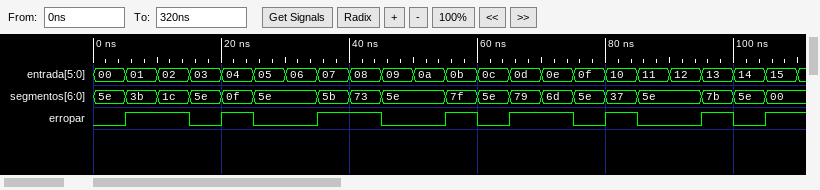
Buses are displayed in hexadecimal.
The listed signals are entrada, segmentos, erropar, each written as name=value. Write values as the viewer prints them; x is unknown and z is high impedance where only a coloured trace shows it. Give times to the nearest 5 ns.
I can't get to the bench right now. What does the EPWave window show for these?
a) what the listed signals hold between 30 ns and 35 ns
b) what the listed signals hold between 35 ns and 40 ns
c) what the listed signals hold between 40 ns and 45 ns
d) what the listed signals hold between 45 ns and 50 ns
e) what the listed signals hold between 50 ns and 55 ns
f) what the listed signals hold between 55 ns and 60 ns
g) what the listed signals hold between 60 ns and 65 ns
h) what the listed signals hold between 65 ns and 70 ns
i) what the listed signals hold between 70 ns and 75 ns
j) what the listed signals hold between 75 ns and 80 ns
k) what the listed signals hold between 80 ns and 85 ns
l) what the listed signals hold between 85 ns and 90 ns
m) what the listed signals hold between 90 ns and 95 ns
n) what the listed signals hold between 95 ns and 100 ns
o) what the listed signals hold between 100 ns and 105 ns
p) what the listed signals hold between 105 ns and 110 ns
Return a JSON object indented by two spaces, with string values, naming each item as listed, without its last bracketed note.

{
  "what the listed signals hold between 30 ns and 35 ns": "entrada=06, segmentos=5e, erropar=0",
  "what the listed signals hold between 35 ns and 40 ns": "entrada=07, segmentos=5b, erropar=1",
  "what the listed signals hold between 40 ns and 45 ns": "entrada=08, segmentos=73, erropar=1",
  "what the listed signals hold between 45 ns and 50 ns": "entrada=09, segmentos=5e, erropar=0",
  "what the listed signals hold between 50 ns and 55 ns": "entrada=0a, segmentos=5e, erropar=0",
  "what the listed signals hold between 55 ns and 60 ns": "entrada=0b, segmentos=7f, erropar=1",
  "what the listed signals hold between 60 ns and 65 ns": "entrada=0c, segmentos=5e, erropar=0",
  "what the listed signals hold between 65 ns and 70 ns": "entrada=0d, segmentos=79, erropar=1",
  "what the listed signals hold between 70 ns and 75 ns": "entrada=0e, segmentos=6d, erropar=1",
  "what the listed signals hold between 75 ns and 80 ns": "entrada=0f, segmentos=5e, erropar=0",
  "what the listed signals hold between 80 ns and 85 ns": "entrada=10, segmentos=37, erropar=1",
  "what the listed signals hold between 85 ns and 90 ns": "entrada=11, segmentos=5e, erropar=0",
  "what the listed signals hold between 90 ns and 95 ns": "entrada=12, segmentos=5e, erropar=0",
  "what the listed signals hold between 95 ns and 100 ns": "entrada=13, segmentos=7b, erropar=1",
  "what the listed signals hold between 100 ns and 105 ns": "entrada=14, segmentos=5e, erropar=0",
  "what the listed signals hold between 105 ns and 110 ns": "entrada=15, segmentos=00, erropar=1"
}
